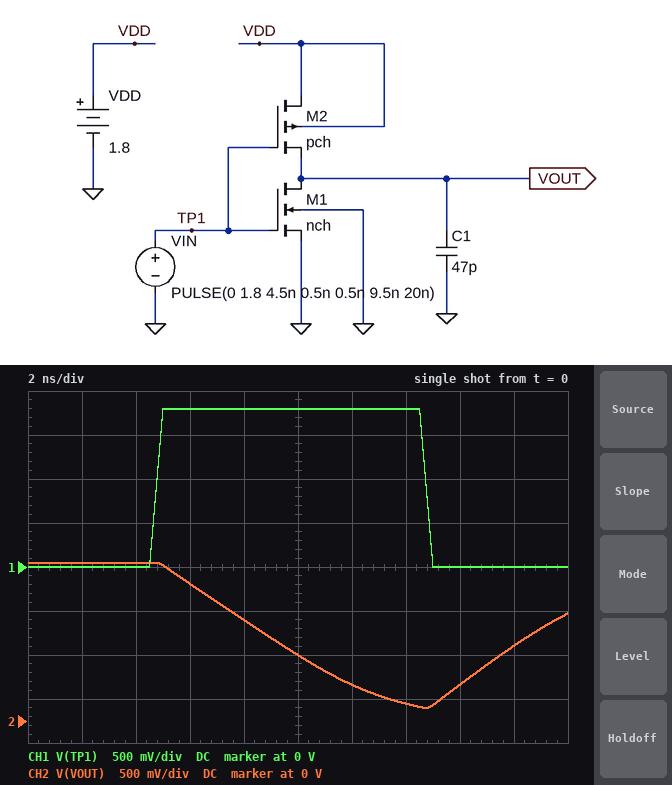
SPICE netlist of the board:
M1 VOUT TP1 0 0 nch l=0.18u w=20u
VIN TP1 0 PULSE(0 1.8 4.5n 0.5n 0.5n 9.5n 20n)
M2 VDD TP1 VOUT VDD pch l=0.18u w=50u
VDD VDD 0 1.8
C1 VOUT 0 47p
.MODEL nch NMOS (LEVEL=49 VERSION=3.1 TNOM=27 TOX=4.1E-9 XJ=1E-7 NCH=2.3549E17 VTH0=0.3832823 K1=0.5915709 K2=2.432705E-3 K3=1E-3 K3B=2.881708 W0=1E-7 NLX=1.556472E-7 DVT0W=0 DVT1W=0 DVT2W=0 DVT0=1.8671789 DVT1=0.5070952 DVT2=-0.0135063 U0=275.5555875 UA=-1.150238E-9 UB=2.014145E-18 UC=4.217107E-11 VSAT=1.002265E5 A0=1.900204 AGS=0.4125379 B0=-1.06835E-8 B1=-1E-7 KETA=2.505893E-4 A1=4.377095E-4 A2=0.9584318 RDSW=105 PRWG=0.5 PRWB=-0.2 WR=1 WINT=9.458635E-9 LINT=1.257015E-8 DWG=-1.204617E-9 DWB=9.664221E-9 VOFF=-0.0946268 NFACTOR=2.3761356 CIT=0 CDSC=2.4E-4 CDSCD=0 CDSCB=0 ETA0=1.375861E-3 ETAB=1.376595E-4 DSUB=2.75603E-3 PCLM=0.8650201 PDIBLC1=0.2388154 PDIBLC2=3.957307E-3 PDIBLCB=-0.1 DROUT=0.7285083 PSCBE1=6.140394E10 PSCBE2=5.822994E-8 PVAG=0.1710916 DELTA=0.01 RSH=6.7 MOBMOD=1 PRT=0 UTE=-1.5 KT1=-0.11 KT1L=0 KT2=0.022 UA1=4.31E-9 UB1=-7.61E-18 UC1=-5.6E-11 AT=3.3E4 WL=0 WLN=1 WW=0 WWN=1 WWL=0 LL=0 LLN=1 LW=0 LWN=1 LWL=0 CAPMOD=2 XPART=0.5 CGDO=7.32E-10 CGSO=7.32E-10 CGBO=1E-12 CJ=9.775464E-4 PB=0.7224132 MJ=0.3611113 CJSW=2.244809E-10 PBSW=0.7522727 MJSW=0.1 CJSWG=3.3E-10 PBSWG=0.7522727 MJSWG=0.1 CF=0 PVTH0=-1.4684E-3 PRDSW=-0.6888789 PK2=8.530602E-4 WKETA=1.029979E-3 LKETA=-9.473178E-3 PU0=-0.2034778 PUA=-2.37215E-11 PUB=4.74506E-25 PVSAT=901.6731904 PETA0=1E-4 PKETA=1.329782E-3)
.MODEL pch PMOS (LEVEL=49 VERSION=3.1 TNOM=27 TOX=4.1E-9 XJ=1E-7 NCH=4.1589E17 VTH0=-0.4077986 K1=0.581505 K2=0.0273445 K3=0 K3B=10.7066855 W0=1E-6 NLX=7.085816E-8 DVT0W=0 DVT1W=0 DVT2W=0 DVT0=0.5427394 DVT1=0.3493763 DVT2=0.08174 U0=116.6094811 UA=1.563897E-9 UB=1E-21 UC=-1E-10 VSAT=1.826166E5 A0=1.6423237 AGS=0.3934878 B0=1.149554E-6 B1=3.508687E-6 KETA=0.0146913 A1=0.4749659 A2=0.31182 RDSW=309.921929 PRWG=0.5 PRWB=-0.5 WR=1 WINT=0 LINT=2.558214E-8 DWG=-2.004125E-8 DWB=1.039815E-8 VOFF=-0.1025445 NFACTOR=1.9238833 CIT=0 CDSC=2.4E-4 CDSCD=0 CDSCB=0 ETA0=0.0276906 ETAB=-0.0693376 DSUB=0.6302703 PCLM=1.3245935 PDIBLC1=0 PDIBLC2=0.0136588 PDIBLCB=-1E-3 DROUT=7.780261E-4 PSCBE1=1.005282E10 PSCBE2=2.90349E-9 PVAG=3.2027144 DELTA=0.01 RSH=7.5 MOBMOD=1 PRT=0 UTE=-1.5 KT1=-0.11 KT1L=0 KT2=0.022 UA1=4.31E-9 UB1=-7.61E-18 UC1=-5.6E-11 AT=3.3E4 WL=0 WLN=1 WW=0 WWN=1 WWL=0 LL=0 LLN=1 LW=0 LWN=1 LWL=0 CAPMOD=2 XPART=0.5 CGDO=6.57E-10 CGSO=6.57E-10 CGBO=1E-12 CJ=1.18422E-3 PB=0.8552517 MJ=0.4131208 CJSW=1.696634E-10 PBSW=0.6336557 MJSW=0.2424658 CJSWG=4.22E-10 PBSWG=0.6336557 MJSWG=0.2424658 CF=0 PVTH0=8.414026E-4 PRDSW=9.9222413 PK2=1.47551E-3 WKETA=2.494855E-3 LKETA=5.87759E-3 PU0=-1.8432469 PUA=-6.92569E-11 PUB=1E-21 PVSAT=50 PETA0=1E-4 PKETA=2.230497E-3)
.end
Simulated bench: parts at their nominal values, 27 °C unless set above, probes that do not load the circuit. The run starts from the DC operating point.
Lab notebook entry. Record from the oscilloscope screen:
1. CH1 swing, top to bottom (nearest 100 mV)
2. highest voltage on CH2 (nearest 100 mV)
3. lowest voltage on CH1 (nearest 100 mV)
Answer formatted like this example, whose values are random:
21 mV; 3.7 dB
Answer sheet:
1.8 V; 1.8 V; 0 V
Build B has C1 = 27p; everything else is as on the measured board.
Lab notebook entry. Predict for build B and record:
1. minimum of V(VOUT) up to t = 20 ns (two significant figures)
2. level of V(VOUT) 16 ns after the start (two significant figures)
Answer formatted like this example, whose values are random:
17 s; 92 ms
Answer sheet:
5.5 mV; 470 mV
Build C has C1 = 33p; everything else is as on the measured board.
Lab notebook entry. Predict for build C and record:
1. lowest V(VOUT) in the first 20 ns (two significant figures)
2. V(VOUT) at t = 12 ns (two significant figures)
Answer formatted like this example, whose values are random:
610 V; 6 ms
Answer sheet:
25 mV; 130 mV
